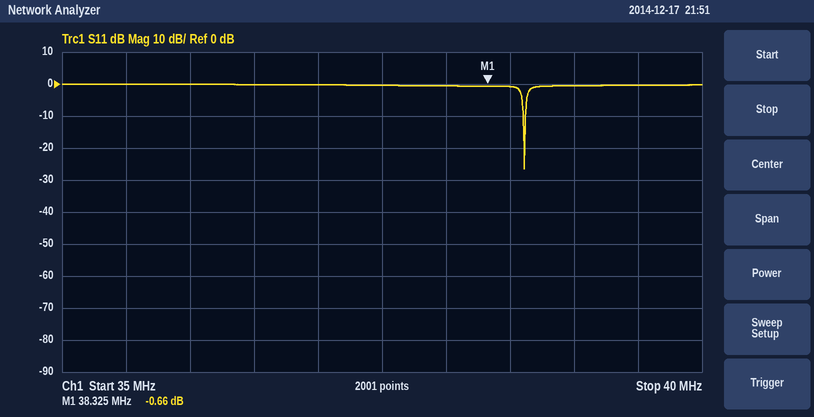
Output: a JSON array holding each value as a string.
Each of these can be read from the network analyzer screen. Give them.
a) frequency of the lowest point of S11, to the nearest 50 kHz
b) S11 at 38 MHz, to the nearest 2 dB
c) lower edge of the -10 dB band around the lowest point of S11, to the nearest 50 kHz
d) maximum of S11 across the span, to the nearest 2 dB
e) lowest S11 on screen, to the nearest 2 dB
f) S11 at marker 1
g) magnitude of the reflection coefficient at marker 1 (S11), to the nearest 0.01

["38.60 MHz", "0 dB", "38.60 MHz", "0 dB", "-26 dB", "-0.66 dB", "0.93"]
